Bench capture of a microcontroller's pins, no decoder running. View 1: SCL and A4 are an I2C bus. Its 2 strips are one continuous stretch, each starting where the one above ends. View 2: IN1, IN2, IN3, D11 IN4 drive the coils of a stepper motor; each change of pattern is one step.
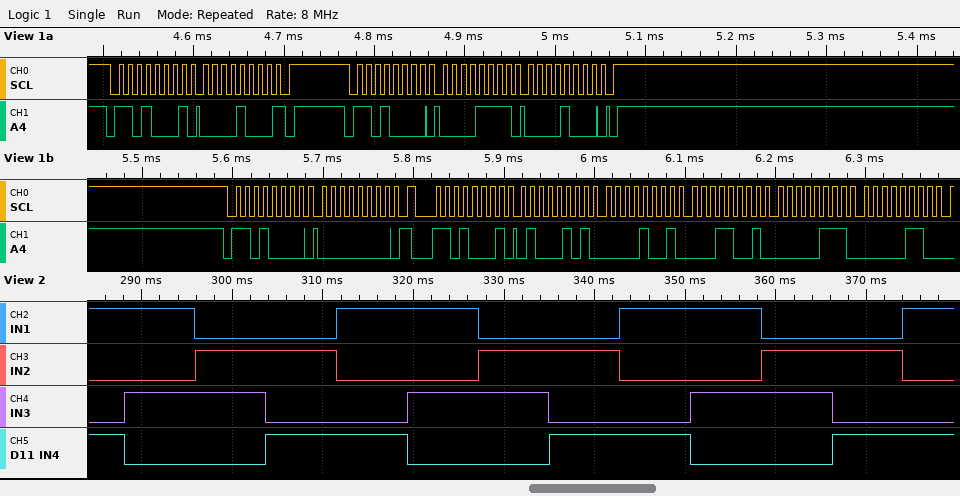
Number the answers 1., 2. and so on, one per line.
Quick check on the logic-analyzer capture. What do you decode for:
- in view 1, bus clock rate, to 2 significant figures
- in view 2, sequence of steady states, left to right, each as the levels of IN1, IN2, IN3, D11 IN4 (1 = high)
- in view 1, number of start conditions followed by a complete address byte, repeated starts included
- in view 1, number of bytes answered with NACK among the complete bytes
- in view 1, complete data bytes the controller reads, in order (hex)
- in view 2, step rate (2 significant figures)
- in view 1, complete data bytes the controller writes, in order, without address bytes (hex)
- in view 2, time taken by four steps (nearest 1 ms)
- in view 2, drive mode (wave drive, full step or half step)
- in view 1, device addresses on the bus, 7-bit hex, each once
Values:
1. 100 kHz
2. 1001 1010 0110 0101 1001 1010 0110 0101 1001 1010 0110 0101 1001
3. 4
4. 1
5. 08 45 09 19 07 06
6. 130 steps/s
7. 0F 08 00
8. 31 ms
9. full step
10. 0x68
